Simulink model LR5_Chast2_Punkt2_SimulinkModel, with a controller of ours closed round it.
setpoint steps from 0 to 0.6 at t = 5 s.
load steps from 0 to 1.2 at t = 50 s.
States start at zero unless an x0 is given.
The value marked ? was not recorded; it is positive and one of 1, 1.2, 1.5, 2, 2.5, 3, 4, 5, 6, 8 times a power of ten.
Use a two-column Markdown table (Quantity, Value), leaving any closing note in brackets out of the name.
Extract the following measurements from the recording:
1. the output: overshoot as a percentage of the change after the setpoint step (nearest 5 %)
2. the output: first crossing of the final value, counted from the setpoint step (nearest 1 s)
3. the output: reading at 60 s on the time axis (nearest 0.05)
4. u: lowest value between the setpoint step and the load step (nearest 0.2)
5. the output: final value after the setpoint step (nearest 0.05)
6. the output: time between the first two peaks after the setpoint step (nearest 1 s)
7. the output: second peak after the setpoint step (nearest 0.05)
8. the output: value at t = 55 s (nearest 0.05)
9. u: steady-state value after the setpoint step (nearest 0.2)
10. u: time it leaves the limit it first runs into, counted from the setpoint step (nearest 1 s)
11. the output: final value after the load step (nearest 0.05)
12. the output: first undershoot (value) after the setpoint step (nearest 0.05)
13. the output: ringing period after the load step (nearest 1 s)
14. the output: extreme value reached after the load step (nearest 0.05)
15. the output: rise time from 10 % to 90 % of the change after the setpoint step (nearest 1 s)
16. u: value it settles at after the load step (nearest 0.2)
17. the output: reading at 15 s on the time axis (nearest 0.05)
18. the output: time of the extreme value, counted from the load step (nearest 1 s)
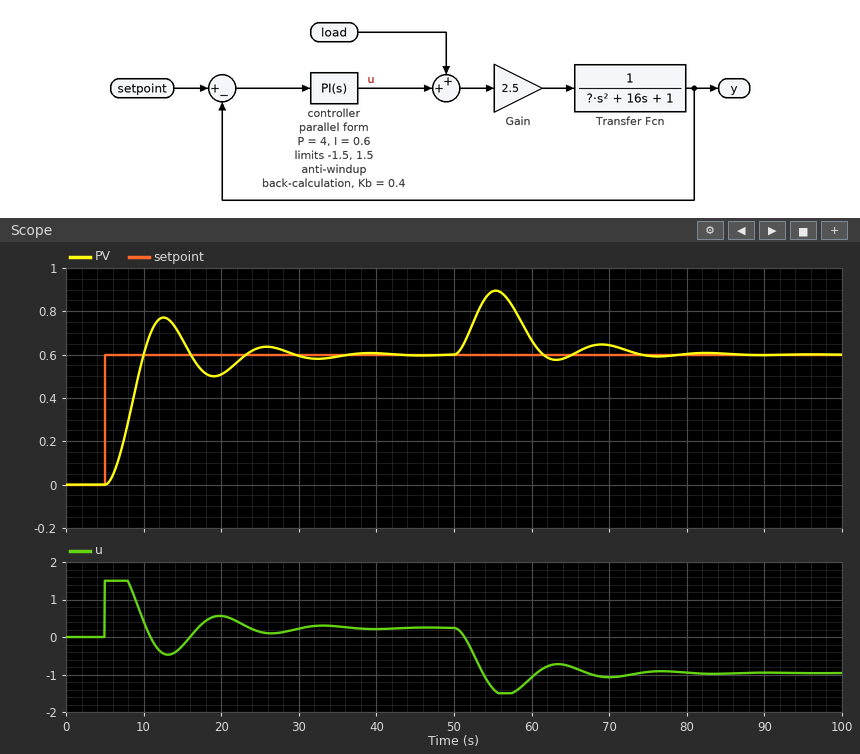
| Quantity | Value |
|---|---|
| the output: overshoot as a percentage of the change after the setpoint step | 30 % |
| the output: first crossing of the final value, counted from the setpoint step | 5 s |
| the output: reading at 60 s on the time axis | 0.65 |
| u: lowest value between the setpoint step and the load step | -0.4 |
| the output: final value after the setpoint step | 0.60 |
| the output: time between the first two peaks after the setpoint step | 13 s |
| the output: second peak after the setpoint step | 0.65 |
| the output: value at t = 55 s | 0.90 |
| u: steady-state value after the setpoint step | 0.2 |
| u: time it leaves the limit it first runs into, counted from the setpoint step | 3 s |
| the output: final value after the load step | 0.60 |
| the output: first undershoot (value) after the setpoint step | 0.50 |
| the output: ringing period after the load step | 14 s |
| the output: extreme value reached after the load step | 0.90 |
| the output: rise time from 10 % to 90 % of the change after the setpoint step | 3 s |
| u: value it settles at after the load step | -1.0 |
| the output: reading at 15 s on the time axis | 0.65 |
| the output: time of the extreme value, counted from the load step | 5 s |
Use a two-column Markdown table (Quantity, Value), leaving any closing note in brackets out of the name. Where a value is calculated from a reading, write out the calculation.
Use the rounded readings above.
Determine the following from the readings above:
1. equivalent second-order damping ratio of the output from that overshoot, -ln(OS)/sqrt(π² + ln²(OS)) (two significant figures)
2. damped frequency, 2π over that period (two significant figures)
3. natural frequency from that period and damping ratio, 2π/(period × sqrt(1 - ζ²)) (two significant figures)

| Quantity | Value |
|---|---|
| equivalent second-order damping ratio of the output from that overshoot, -ln(OS)/sqrt(π² + ln²(OS)) | ln(0.3) = -1.204; 1.204 / sqrt(9.870 + 1.450) = 0.36 |
| damped frequency, 2π over that period | 2π / 13 = 0.48 rad/s |
| natural frequency from that period and damping ratio, 2π/(period × sqrt(1 - ζ²)) | 2π / (13 × sqrt(1 - 0.36²)) = 0.52 rad/s |
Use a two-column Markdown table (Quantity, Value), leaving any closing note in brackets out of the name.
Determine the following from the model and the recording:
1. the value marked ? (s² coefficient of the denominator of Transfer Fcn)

| Quantity | Value |
|---|---|
| the value marked ? | 40 |
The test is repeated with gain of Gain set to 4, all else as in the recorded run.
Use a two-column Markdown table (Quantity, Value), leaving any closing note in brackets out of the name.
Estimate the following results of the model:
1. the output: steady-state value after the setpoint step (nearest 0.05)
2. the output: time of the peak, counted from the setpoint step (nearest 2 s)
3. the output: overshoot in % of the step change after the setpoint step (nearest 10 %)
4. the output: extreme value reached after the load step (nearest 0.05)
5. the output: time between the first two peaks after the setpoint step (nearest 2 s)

| Quantity | Value |
|---|---|
| the output: steady-state value after the setpoint step | 0.60 |
| the output: time of the peak, counted from the setpoint step | 6 s |
| the output: overshoot in % of the step change after the setpoint step | 40 % |
| the output: extreme value reached after the load step | 0.95 |
| the output: time between the first two peaks after the setpoint step | 10 s |
